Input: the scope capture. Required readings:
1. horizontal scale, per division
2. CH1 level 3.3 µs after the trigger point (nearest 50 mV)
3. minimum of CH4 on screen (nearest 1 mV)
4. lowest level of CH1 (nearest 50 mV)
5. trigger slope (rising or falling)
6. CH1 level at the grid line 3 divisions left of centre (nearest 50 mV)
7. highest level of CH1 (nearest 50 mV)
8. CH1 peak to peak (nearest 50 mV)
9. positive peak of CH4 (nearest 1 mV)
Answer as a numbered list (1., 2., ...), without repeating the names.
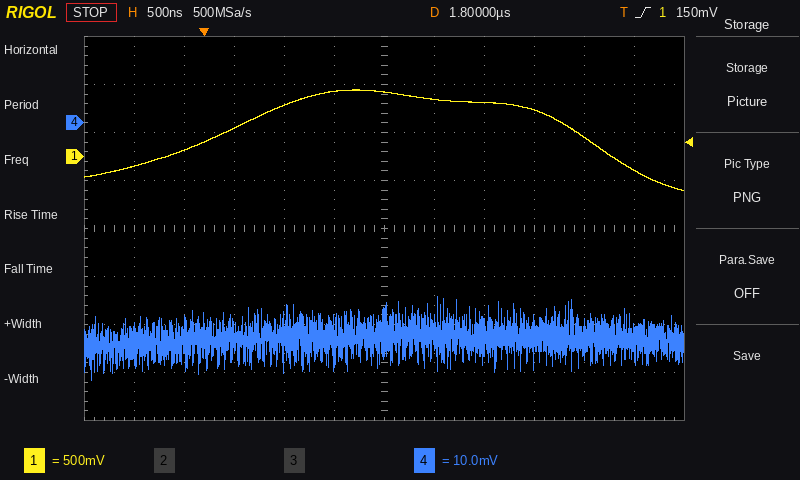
1. 500 ns
2. 500 mV
3. -54 mV
4. -350 mV
5. rising
6. 300 mV
7. 700 mV
8. 1.05 V
9. -36 mV
